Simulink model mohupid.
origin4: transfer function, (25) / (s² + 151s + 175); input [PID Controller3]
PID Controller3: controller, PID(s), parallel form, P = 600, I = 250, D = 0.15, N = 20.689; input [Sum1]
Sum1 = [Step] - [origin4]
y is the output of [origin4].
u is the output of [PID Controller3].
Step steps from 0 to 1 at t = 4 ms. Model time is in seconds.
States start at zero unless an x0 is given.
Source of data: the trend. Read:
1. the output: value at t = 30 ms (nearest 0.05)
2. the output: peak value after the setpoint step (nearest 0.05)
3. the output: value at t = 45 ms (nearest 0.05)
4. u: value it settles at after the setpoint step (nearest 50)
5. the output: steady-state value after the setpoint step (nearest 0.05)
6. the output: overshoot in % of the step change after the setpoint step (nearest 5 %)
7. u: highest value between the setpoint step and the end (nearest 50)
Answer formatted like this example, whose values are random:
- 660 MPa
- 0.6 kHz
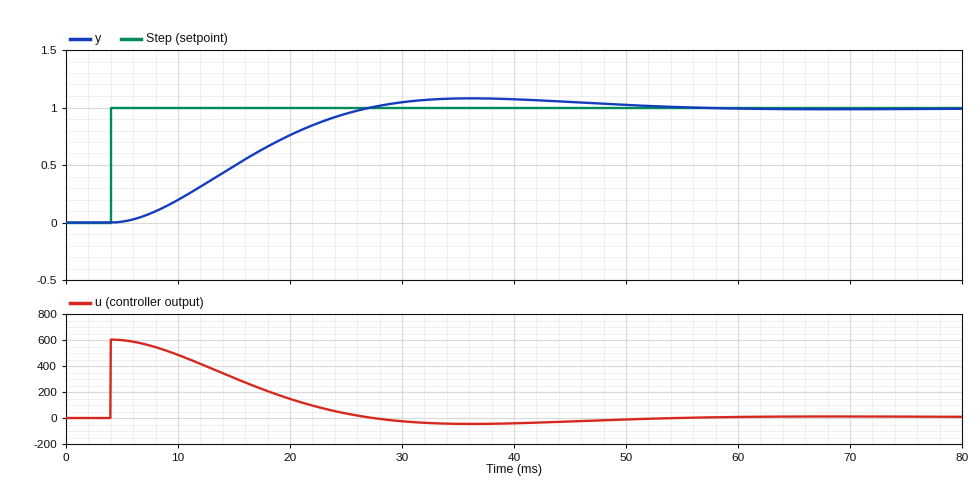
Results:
- 1.05
- 1.10
- 1.05
- 0
- 1.00
- 10 %
- 600
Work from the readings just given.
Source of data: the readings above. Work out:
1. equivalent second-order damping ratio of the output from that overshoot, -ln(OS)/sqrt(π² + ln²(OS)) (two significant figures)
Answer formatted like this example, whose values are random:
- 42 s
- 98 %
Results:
- 0.59
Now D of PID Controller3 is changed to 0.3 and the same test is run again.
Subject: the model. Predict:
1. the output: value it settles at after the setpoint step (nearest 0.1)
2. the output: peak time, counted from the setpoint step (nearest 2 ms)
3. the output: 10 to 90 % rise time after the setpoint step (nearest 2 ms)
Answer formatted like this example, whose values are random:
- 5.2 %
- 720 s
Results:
- 1.0
- 32 ms
- 16 ms
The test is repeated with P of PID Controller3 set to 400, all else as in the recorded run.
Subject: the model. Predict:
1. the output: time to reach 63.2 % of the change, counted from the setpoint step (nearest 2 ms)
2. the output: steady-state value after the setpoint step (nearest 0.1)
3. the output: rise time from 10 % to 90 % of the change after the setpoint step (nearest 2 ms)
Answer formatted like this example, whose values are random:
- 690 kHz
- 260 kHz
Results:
- 18 ms
- 1.0
- 22 ms
